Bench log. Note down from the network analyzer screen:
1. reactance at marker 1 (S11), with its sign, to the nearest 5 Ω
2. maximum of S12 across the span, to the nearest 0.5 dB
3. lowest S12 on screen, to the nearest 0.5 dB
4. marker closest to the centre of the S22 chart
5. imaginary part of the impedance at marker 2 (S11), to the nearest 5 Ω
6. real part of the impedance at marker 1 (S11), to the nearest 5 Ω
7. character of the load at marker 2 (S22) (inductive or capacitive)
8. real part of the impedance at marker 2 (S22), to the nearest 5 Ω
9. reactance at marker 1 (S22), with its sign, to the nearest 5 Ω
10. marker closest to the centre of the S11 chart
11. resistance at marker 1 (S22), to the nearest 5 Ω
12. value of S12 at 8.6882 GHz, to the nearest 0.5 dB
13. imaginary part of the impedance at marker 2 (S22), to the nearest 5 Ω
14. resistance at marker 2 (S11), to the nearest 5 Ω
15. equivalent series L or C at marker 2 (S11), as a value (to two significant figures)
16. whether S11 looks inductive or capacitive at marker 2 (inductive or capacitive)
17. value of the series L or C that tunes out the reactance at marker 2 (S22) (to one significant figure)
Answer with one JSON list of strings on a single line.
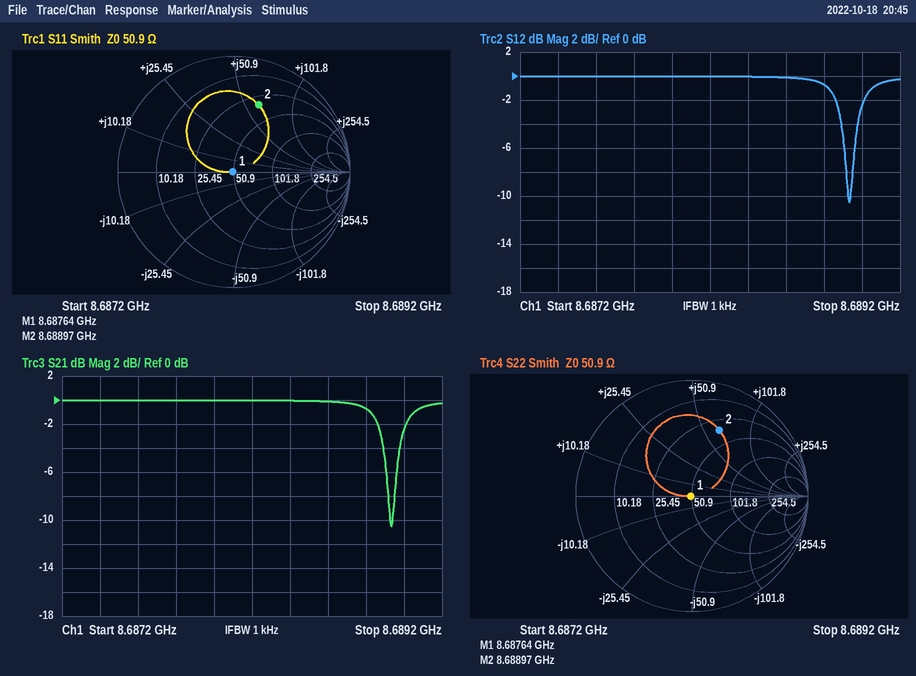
["0 Ω", "0.0 dB", "-10.5 dB", "marker 1", "+60 Ω", "50 Ω", "inductive", "35 Ω", "0 Ω", "marker 1", "50 Ω", "0.0 dB", "+65 Ω", "35 Ω", "1.1 nH", "inductive", "300 fF"]
